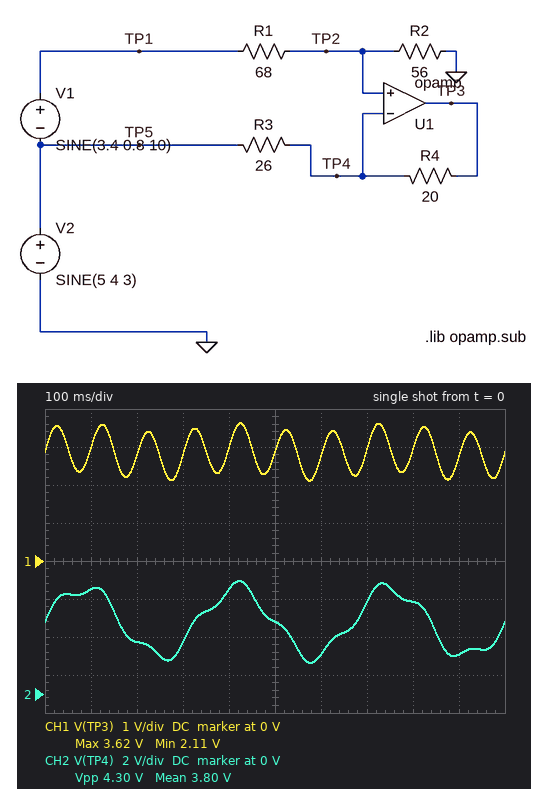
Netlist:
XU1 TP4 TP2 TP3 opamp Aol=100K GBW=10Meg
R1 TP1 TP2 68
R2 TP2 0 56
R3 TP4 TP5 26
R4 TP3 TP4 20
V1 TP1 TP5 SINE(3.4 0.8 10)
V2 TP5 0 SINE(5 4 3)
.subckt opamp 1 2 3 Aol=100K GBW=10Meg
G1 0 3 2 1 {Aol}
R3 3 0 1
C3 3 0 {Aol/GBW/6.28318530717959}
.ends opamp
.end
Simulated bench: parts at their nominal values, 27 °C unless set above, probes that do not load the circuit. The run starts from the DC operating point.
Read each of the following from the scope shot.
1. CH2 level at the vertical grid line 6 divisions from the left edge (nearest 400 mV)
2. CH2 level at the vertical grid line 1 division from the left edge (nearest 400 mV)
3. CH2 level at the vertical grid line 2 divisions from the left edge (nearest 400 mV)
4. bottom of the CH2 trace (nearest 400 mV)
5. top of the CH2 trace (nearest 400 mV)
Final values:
2.0 V
5.6 V
2.8 V
1.6 V
6.0 V
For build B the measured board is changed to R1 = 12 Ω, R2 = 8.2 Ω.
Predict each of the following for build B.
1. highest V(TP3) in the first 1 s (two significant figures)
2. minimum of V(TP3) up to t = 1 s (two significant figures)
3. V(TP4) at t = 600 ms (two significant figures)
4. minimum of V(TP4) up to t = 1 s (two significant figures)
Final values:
3.0 V
1.4 V
1.9 V
1.5 V
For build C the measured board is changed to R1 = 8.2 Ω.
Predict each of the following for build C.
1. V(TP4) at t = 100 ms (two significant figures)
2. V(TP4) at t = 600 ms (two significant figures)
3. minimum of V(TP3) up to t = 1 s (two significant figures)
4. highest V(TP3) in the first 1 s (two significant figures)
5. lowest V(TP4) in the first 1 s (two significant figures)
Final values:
11 V
4.0 V
4.8 V
13 V
3.2 V
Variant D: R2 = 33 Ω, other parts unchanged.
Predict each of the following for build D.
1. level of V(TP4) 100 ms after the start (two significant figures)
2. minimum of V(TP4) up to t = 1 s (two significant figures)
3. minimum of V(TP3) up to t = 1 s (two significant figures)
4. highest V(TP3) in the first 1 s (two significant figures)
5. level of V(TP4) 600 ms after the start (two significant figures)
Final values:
4.0 V
1.2 V
-210 mV
2.2 V
1.5 V
